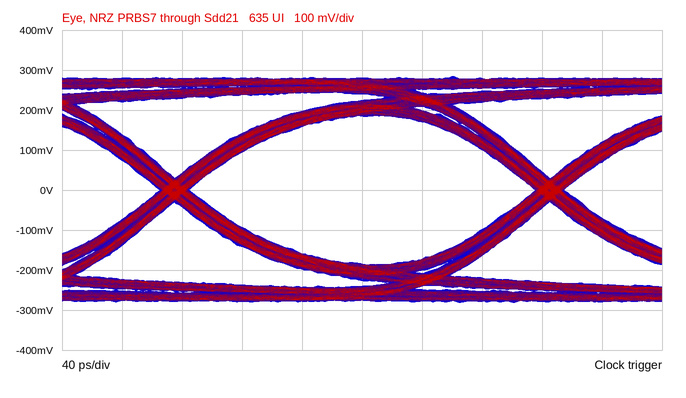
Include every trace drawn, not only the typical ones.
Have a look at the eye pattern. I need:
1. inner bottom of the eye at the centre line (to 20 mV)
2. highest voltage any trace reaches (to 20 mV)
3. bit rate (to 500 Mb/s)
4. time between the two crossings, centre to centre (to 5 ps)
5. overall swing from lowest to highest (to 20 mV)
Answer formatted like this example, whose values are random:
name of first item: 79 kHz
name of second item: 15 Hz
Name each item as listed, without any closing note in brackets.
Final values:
inner bottom of the eye at the centre line: -180 mV
highest voltage any trace reaches: 280 mV
bit rate: 4.0 Gb/s
time between the two crossings, centre to centre: 250 ps
overall swing from lowest to highest: 560 mV
